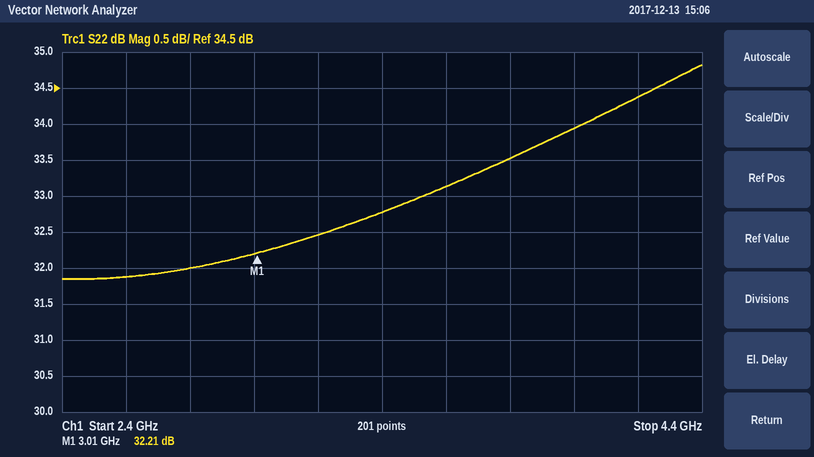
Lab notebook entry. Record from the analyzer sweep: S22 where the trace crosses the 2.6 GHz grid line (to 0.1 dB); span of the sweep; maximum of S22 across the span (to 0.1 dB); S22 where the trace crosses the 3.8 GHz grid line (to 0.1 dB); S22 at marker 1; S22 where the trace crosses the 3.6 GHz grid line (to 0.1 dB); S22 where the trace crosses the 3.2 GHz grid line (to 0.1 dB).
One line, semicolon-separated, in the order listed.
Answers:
31.9 dB; 2 GHz; 34.8 dB; 33.5 dB; 32.21 dB; 33.1 dB; 32.5 dB
